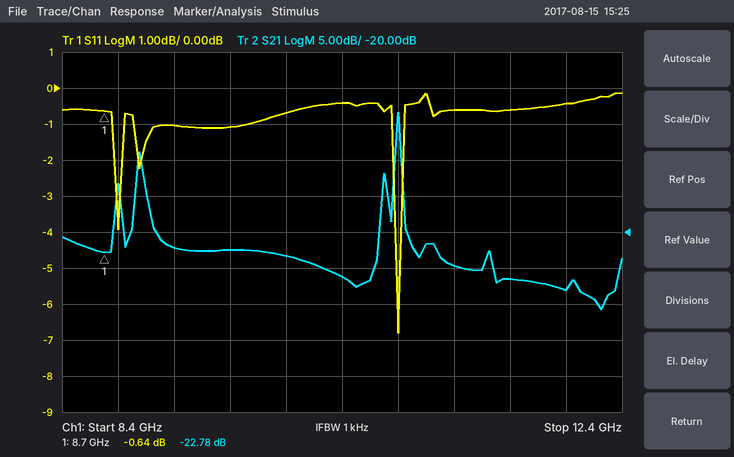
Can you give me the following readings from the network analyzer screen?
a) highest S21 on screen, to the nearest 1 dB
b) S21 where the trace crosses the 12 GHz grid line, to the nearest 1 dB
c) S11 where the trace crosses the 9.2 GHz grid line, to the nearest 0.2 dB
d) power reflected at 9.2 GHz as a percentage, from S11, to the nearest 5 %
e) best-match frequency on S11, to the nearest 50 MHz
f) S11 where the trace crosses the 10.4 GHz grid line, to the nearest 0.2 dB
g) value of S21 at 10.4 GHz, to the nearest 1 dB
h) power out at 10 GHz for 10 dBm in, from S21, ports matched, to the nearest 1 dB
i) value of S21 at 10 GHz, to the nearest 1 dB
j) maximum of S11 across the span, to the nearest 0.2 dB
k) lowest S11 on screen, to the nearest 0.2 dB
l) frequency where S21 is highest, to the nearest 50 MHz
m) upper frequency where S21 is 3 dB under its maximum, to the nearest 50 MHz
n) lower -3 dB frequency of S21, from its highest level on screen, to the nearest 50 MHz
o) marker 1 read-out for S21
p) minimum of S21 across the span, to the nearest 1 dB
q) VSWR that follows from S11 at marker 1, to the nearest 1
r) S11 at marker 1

-3 dB
-28 dB
-1.0 dB
80 %
10.80 GHz
-0.4 dB
-26 dB
-13 dBm
-23 dB
-0.2 dB
-6.8 dB
10.80 GHz
10.80 GHz
10.80 GHz
-22.78 dB
-31 dB
27
-0.64 dB
